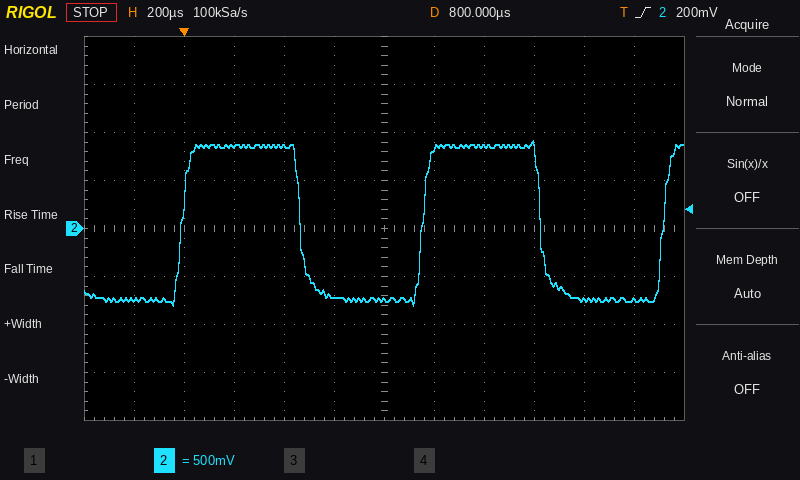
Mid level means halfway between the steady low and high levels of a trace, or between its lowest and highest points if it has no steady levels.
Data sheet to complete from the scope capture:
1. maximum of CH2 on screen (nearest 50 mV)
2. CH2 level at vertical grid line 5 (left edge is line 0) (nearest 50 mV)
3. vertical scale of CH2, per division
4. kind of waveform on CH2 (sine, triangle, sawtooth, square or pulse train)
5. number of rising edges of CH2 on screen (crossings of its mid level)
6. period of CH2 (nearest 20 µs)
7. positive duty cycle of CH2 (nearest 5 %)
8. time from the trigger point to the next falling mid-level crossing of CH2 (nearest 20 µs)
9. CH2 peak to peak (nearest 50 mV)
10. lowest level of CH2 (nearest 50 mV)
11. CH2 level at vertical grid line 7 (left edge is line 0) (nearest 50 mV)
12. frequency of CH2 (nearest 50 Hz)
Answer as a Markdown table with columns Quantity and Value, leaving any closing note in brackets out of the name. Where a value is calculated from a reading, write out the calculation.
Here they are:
| Quantity | Value |
|---|---|
| maximum of CH2 on screen | 900 mV |
| CH2 level at vertical grid line 5 (left edge is line 0) | -700 mV |
| vertical scale of CH2, per division | 500 mV |
| kind of waveform on CH2 | square |
| number of rising edges of CH2 on screen | 3 |
| period of CH2 | 960 µs |
| positive duty cycle of CH2 | 50 % |
| time from the trigger point to the next falling mid-level crossing of CH2 | 460 µs |
| CH2 peak to peak | 900 mV − (-800 mV) = 1.70 V |
| lowest level of CH2 | -800 mV |
| CH2 level at vertical grid line 7 (left edge is line 0) | 850 mV |
| frequency of CH2 | 1 / 960 µs ≈ 1.04 kHz, so 1.05 kHz to the nearest 50 Hz |
